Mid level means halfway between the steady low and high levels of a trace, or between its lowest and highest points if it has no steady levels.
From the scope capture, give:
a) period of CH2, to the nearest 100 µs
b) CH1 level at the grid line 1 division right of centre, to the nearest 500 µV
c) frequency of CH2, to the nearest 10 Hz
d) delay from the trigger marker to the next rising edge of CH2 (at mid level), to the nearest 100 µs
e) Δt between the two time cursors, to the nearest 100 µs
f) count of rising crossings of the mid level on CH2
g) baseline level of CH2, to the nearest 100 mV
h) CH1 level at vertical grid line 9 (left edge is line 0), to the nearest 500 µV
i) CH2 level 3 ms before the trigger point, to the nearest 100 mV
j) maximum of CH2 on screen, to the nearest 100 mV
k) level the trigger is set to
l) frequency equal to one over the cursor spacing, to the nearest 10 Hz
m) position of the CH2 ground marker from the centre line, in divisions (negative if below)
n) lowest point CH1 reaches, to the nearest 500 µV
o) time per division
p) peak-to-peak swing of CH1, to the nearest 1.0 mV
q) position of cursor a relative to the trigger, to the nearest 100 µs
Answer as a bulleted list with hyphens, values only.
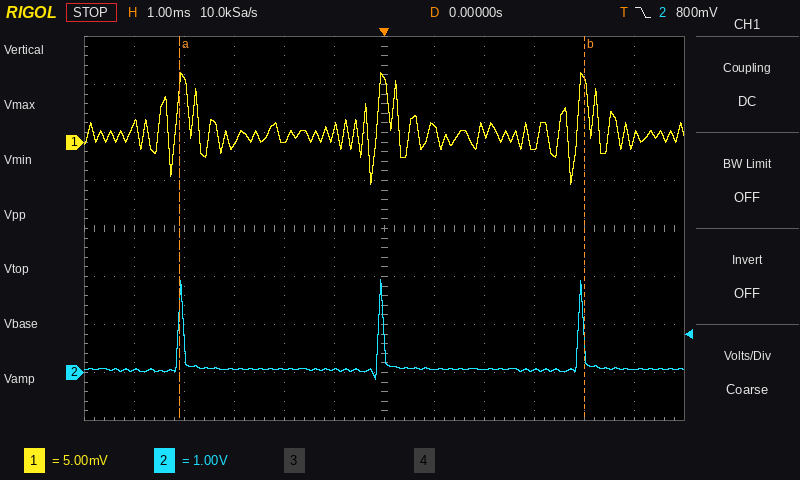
- 4.0 ms
- 1.5 mV
- 250 Hz
- 3.9 ms
- 8.1 ms
- 3
- 100 mV
- -500 µV
- 100 mV
- 1.9 V
- 800 mV
- 120 Hz
- -3.0 div
- -4.5 mV
- 1 ms
- 12.0 mV
- -4.1 ms
